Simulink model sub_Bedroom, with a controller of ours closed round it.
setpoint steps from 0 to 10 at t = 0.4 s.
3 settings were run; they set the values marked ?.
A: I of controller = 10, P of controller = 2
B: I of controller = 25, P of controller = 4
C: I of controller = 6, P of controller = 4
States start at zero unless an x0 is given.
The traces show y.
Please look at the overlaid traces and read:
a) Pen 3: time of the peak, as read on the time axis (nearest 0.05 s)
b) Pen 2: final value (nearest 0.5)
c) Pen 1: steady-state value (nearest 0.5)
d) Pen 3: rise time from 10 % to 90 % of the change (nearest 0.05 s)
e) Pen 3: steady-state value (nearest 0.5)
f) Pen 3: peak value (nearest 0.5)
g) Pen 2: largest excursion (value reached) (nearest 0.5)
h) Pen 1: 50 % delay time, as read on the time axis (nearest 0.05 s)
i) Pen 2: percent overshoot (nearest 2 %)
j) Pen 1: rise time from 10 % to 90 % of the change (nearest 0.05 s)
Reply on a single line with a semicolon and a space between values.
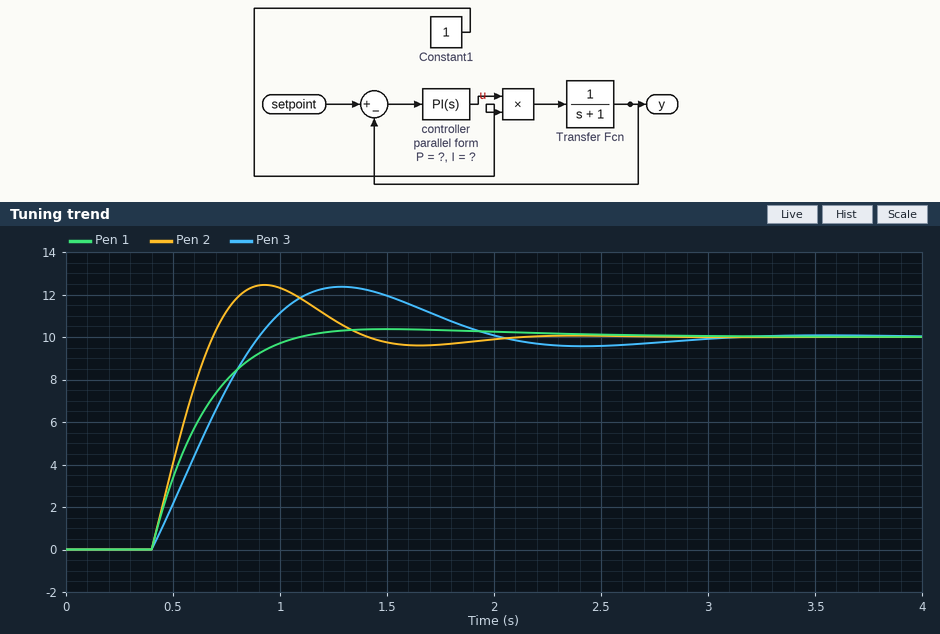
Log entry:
1.30 s; 10.0; 10.0; 0.40 s; 10.0; 12.5; 12.5; 0.55 s; 24 %; 0.45 s
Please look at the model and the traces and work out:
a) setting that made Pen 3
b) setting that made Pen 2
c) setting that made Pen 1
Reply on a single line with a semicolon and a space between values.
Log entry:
A; B; C
